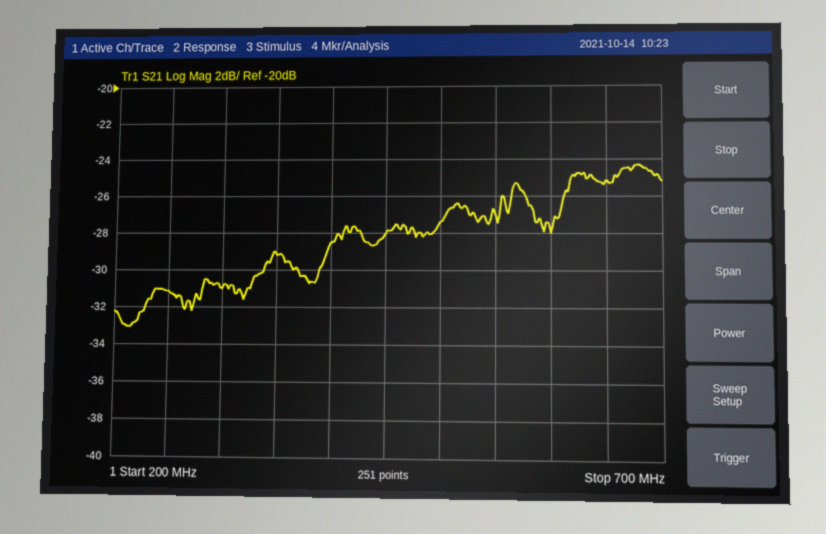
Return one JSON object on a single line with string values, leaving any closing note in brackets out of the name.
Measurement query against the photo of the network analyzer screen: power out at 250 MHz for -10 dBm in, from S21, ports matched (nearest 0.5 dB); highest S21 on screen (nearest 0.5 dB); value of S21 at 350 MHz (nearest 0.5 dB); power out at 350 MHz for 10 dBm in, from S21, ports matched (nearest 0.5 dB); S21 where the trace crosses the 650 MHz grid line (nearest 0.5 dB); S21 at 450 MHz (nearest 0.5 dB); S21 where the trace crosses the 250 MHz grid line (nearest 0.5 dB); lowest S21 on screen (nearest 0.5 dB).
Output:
{"power out at 250 MHz for -10 dBm in, from S21, ports matched": "-41.0 dBm", "highest S21 on screen": "-24.5 dB", "value of S21 at 350 MHz": "-29.0 dB", "power out at 350 MHz for 10 dBm in, from S21, ports matched": "-19.0 dBm", "S21 where the trace crosses the 650 MHz grid line": "-25.0 dB", "S21 at 450 MHz": "-28.0 dB", "S21 where the trace crosses the 250 MHz grid line": "-31.0 dB", "lowest S21 on screen": "-33.0 dB"}
